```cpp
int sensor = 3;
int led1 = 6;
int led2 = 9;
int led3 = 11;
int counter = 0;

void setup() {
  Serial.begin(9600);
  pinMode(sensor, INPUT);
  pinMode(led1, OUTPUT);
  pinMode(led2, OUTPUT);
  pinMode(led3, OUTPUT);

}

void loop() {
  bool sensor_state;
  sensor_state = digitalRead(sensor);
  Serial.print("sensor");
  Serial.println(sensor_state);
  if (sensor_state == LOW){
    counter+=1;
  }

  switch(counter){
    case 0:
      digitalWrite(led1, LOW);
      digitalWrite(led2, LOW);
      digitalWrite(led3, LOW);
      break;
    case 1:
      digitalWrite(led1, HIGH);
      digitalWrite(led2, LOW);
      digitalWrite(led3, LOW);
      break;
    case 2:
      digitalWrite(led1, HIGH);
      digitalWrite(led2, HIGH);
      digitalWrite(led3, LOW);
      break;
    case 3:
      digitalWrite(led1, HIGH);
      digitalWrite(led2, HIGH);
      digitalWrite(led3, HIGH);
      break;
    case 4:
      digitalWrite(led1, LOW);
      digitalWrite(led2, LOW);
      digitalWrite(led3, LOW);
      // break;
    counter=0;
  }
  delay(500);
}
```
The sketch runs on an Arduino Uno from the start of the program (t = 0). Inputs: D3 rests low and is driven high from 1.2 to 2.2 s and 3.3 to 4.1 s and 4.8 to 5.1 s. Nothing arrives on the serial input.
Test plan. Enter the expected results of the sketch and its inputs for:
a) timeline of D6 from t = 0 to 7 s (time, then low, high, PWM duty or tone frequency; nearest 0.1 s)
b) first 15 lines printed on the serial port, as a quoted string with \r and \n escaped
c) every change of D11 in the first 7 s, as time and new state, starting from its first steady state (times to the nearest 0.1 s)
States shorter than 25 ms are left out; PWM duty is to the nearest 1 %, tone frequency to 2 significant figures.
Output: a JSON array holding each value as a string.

["0 s high; 2.5 s low; 3 s high; 6 s low; 6.5 s high", "\"sensor0\\r\\nsensor0\\r\\nsensor0\\r\\nsensor1\\r\\nsensor1\\r\\nsensor0\\r\\nsensor0\\r\\nsensor1\\r\\nsensor1\\r\\nsensor0\\r\\nsensor1\\r\\nsensor0\\r\\nsensor0\\r\\nsensor0\\r\\nsensor0\\r\\n\"", "0 s low; 1 s high; 2.5 s low; 5.5 s high; 6 s low"]
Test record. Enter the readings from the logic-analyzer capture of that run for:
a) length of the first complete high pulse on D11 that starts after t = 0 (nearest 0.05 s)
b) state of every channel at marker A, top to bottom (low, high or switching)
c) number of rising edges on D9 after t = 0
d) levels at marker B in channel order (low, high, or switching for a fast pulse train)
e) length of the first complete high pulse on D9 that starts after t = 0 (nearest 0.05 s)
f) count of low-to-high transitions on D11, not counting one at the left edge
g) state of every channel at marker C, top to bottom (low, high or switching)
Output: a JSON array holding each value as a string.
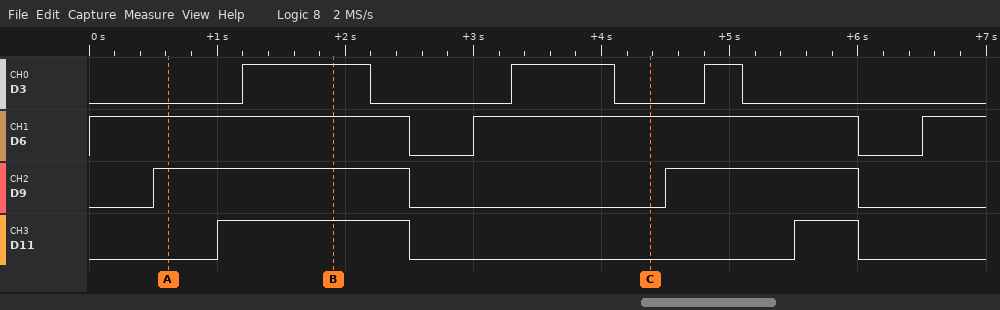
["1.50 s", "D3 low, D6 high, D9 high, D11 low", "2", "D3 high, D6 high, D9 high, D11 high", "2.00 s", "2", "D3 low, D6 high, D9 low, D11 low"]
